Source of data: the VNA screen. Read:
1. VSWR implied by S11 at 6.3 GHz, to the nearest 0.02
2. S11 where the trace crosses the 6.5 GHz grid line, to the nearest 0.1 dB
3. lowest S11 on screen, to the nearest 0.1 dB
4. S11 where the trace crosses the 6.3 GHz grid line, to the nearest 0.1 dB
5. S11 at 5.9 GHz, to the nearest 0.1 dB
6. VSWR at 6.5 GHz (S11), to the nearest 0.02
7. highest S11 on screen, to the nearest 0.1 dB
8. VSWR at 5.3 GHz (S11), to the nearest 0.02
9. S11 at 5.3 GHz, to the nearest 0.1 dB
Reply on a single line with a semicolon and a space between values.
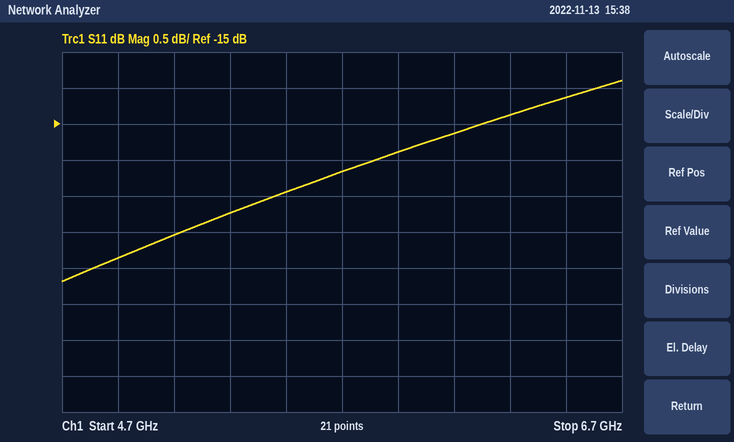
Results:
1.44; -14.6 dB; -17.2 dB; -14.9 dB; -15.4 dB; 1.46; -14.4 dB; 1.36; -16.2 dB
